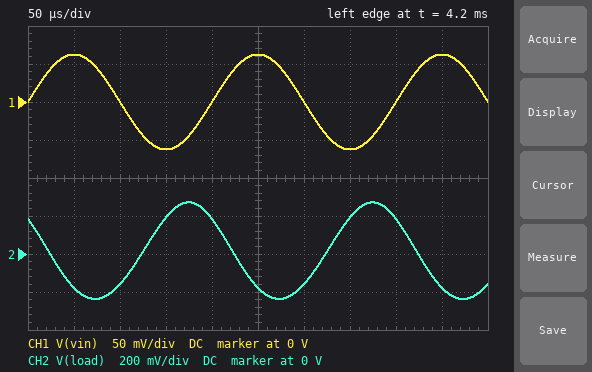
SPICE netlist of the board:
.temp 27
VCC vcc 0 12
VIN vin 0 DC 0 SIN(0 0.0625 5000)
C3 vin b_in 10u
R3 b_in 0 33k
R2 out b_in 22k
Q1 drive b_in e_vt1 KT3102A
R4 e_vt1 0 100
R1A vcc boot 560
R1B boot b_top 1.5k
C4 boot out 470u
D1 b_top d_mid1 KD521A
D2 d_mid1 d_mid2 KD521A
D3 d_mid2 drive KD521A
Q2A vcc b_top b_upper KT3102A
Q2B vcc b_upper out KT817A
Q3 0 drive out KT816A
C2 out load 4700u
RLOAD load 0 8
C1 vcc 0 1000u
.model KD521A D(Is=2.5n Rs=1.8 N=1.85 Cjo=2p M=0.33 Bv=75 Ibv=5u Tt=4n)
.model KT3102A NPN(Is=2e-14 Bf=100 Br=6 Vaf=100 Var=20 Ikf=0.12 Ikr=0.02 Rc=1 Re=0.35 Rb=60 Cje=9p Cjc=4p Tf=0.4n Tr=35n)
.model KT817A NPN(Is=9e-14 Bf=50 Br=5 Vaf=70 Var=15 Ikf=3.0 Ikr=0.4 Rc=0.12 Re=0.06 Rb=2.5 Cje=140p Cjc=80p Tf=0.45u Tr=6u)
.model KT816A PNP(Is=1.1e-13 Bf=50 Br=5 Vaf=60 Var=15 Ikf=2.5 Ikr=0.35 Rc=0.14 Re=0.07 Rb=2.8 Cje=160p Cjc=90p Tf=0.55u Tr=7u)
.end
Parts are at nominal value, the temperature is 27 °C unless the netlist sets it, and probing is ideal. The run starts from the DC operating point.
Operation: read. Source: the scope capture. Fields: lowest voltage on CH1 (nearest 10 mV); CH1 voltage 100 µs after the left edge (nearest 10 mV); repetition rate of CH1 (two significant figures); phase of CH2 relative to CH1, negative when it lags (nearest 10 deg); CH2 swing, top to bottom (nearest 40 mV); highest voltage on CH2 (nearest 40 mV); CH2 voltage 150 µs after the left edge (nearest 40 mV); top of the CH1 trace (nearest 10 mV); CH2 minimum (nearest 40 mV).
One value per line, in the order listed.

-60 mV
0 V
5.0 kHz
140 deg
520 mV
280 mV
200 mV
60 mV
-240 mV
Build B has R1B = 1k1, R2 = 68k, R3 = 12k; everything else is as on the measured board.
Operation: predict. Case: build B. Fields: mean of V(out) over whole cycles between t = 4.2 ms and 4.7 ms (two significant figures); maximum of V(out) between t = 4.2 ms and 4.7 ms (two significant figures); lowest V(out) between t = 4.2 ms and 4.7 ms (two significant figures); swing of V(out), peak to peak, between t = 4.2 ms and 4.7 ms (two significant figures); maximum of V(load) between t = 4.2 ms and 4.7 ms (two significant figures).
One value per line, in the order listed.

7.6 V
8.1 V
7.3 V
840 mV
620 mV
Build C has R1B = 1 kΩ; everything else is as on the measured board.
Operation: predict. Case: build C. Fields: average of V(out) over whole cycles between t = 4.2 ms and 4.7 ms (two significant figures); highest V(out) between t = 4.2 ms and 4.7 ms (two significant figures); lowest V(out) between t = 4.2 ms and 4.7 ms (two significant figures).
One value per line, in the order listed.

3.7 V
3.9 V
3.4 V
